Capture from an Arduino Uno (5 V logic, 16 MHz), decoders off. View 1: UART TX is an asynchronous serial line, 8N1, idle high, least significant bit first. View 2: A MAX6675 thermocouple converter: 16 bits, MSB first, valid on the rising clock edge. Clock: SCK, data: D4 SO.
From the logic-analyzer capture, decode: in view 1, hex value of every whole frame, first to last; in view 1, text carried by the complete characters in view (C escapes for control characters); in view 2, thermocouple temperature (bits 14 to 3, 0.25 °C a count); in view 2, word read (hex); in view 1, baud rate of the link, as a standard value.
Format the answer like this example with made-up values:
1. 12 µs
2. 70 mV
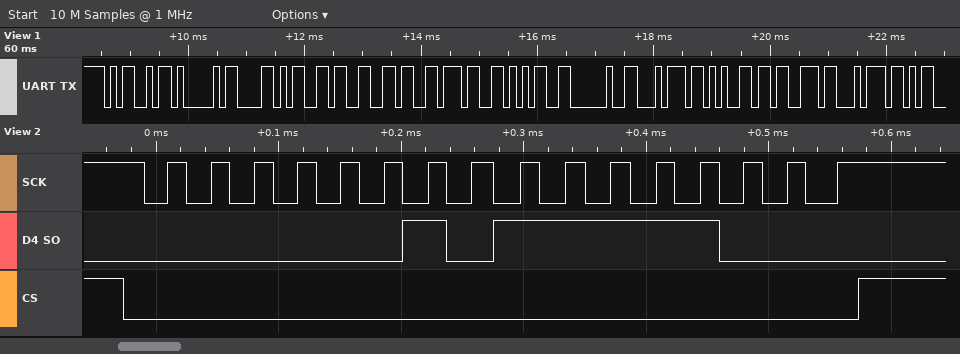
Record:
1. 4D 41 58 36 36 37 35 20 74 65 73 74
2. "MAX6675 test"
3. 23.75 °C
4. 0x02F8
5. 9600 baud
